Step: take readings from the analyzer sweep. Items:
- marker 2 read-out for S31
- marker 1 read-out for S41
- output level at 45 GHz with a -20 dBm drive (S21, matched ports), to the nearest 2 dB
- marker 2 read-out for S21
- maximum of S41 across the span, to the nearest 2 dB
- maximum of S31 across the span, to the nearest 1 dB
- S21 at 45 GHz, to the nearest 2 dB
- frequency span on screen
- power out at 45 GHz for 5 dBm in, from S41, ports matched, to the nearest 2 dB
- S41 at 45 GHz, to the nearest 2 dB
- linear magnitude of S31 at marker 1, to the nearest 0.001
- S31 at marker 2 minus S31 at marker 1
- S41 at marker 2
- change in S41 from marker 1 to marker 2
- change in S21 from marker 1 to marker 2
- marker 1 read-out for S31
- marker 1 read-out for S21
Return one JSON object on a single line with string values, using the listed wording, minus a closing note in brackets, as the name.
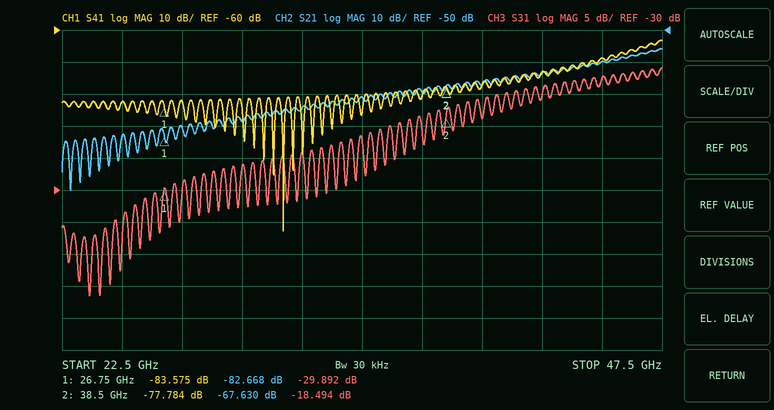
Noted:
{"marker 2 read-out for S31": "-18.494 dB", "marker 1 read-out for S41": "-83.575 dB", "output level at 45 GHz with a -20 dBm drive (S21, matched ports), to the nearest 2 dB": "-80 dBm", "marker 2 read-out for S21": "-67.630 dB", "maximum of S41 across the span, to the nearest 2 dB": "-64 dB", "maximum of S31 across the span, to the nearest 1 dB": "-11 dB", "S21 at 45 GHz, to the nearest 2 dB": "-60 dB", "frequency span on screen": "25 GHz", "power out at 45 GHz for 5 dBm in, from S41, ports matched, to the nearest 2 dB": "-64 dBm", "S41 at 45 GHz, to the nearest 2 dB": "-68 dB", "linear magnitude of S31 at marker 1, to the nearest 0.001": "0.032", "S31 at marker 2 minus S31 at marker 1": "11.398 dB", "S41 at marker 2": "-77.784 dB", "change in S41 from marker 1 to marker 2": "5.791 dB", "change in S21 from marker 1 to marker 2": "15.038 dB", "marker 1 read-out for S31": "-29.892 dB", "marker 1 read-out for S21": "-82.668 dB"}
